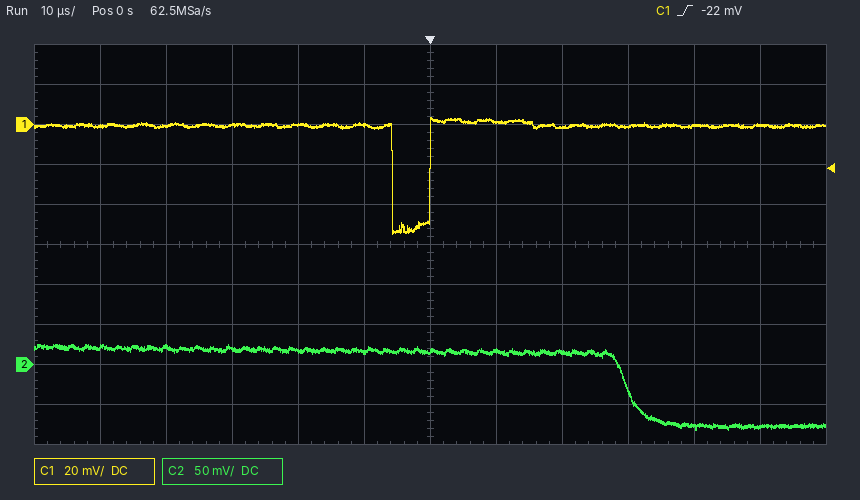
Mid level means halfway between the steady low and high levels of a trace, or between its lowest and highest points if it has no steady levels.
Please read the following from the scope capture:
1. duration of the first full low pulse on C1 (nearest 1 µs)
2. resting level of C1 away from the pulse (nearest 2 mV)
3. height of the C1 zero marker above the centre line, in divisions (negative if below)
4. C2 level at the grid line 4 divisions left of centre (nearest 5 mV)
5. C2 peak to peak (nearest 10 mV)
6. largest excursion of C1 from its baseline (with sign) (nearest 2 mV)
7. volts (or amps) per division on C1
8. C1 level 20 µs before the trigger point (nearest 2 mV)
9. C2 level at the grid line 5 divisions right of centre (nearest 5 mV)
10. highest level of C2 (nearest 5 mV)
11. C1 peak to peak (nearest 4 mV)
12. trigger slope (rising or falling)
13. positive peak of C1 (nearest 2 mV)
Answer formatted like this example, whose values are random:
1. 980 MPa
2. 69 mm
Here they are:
1. 6 µs
2. 0 mV
3. +3.0 div
4. 20 mV
5. 110 mV
6. -54 mV
7. 20 mV
8. 0 mV
9. -80 mV
10. 25 mV
11. 60 mV
12. rising
13. 4 mV
